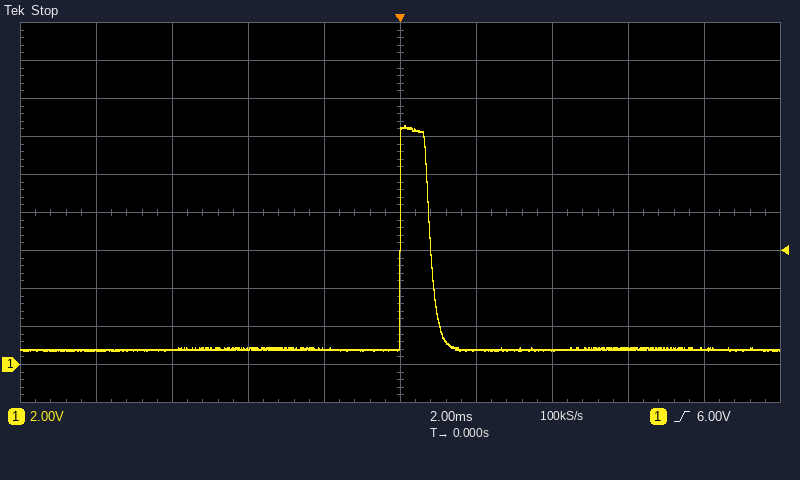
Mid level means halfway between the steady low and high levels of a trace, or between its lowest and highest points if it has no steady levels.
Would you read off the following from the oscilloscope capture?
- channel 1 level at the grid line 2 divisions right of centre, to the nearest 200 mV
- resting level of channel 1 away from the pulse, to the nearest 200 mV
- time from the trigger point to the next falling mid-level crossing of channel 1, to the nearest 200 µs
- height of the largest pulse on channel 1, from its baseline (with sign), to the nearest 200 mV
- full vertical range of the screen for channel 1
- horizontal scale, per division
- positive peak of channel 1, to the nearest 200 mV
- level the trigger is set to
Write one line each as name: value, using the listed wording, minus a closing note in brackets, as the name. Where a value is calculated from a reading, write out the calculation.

channel 1 level at the grid line 2 divisions right of centre, to the nearest 200 mV: 800 mV
resting level of channel 1 away from the pulse, to the nearest 200 mV: 800 mV
time from the trigger point to the next falling mid-level crossing of channel 1, to the nearest 200 µs: 800 µs
height of the largest pulse on channel 1, from its baseline (with sign), to the nearest 200 mV: 12.6 V − (800 mV) = +11.8 V
full vertical range of the screen for channel 1: 20 V
horizontal scale, per division: 2 ms
positive peak of channel 1, to the nearest 200 mV: 12.6 V
level the trigger is set to: 6.00 V
